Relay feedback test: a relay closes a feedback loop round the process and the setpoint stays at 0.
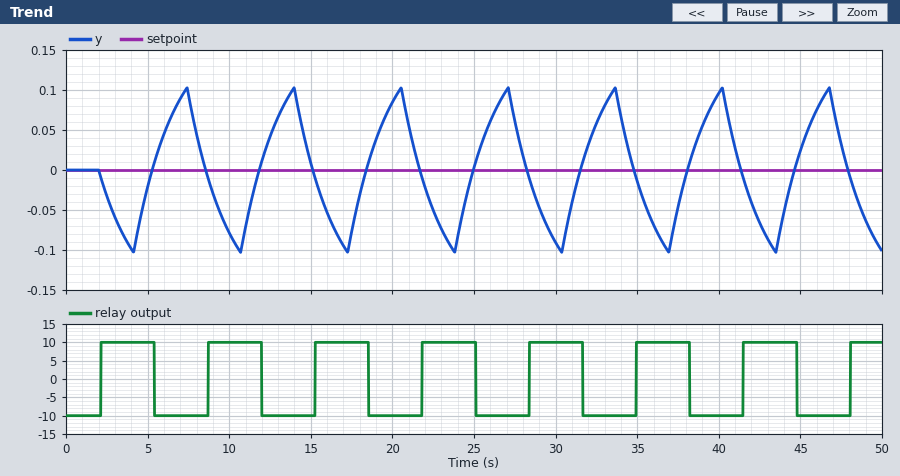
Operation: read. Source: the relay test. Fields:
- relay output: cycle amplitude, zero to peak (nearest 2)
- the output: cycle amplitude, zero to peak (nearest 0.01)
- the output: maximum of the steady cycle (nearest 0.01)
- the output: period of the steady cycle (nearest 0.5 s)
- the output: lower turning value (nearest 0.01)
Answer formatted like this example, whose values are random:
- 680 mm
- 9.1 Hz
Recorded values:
- 10
- 0.10
- 0.10
- 6.5 s
- -0.10
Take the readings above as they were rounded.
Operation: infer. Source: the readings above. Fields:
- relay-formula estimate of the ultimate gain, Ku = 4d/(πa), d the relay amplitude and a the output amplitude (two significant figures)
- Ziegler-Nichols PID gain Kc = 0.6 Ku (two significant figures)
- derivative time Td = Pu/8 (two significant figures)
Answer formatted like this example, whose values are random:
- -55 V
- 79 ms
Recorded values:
- 130
- 78
- 0.81 s
